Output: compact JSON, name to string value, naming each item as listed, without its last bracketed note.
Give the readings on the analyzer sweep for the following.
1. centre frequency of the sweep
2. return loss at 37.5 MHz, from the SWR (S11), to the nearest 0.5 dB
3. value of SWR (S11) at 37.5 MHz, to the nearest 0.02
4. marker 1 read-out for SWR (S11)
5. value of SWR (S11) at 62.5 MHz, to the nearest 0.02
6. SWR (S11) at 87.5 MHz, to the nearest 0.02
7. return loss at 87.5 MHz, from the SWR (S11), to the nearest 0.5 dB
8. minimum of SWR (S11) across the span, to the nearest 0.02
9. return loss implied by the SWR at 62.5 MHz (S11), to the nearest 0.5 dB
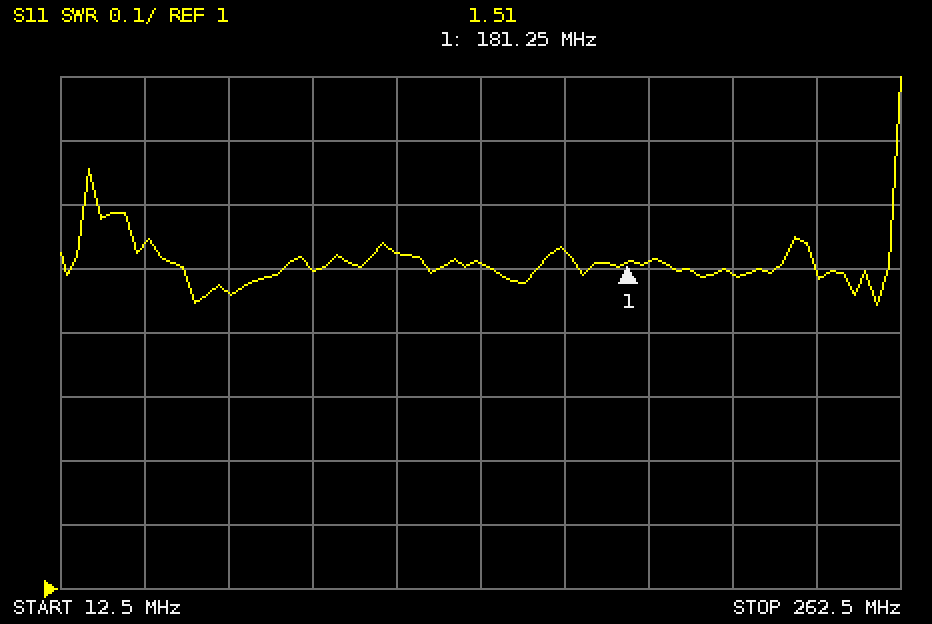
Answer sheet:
{"centre frequency of the sweep": "137.5 MHz", "return loss at 37.5 MHz, from the SWR (S11), to the nearest 0.5 dB": "13.5 dB", "value of SWR (S11) at 37.5 MHz, to the nearest 0.02": "1.54", "marker 1 read-out for SWR": "1.51", "value of SWR (S11) at 62.5 MHz, to the nearest 0.02": "1.46", "SWR (S11) at 87.5 MHz, to the nearest 0.02": "1.50", "return loss at 87.5 MHz, from the SWR (S11), to the nearest 0.5 dB": "14.0 dB", "minimum of SWR (S11) across the span, to the nearest 0.02": "1.44", "return loss implied by the SWR at 62.5 MHz (S11), to the nearest 0.5 dB": "14.5 dB"}
